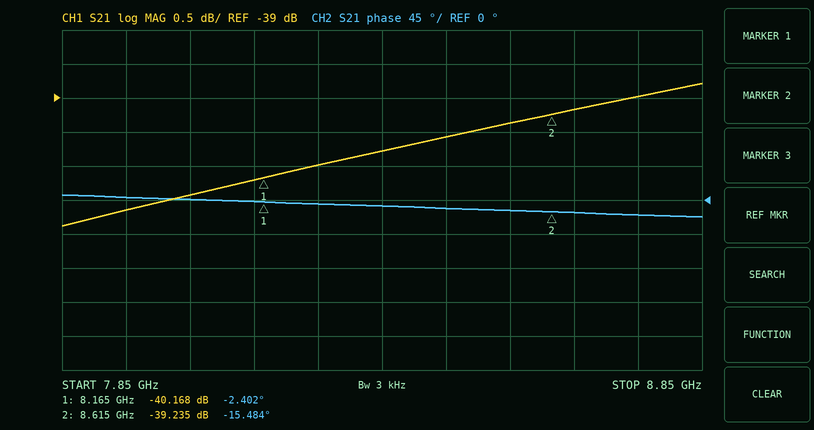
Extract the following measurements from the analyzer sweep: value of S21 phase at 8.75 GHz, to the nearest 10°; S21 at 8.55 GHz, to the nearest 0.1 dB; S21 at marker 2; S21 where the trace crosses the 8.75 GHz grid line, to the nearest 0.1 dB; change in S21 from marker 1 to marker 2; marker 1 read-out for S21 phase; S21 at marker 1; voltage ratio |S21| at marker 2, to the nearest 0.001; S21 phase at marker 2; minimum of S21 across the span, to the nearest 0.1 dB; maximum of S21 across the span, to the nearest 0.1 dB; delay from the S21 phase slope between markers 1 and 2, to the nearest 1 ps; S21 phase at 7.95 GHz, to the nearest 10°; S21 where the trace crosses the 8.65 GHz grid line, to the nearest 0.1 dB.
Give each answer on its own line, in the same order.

-20°
-39.4 dB
-39.235 dB
-39.0 dB
0.933 dB
-2.402°
-40.168 dB
0.011
-15.484°
-40.9 dB
-38.8 dB
81 ps
0°
-39.2 dB
